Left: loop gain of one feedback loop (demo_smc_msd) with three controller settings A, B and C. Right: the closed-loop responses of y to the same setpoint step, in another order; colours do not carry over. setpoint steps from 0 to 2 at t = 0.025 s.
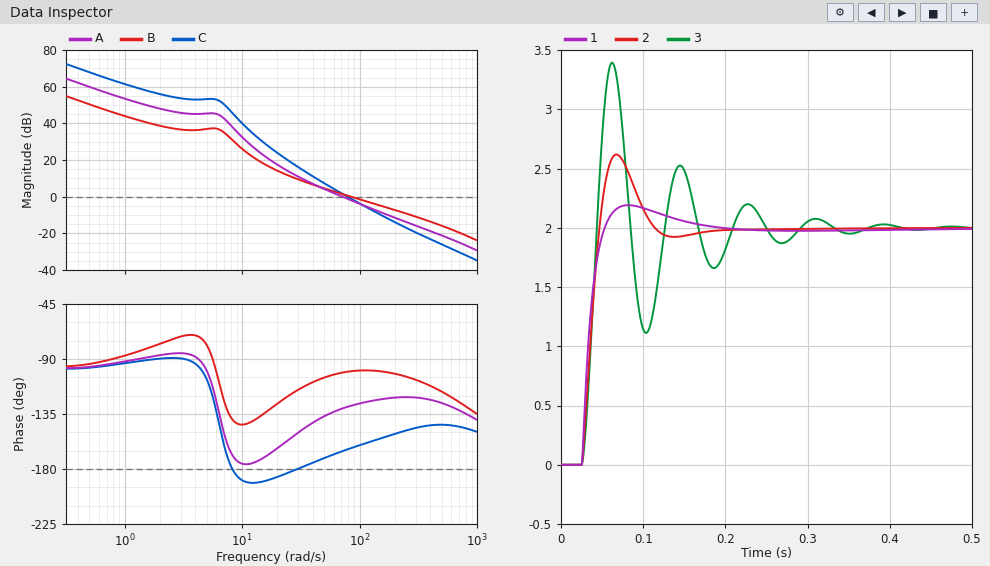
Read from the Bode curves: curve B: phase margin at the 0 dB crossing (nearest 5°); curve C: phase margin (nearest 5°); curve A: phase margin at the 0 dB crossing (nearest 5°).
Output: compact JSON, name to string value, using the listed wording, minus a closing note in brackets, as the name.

{"curve B: phase margin at the 0 dB crossing": "80°", "curve C: phase margin": "15°", "curve A: phase margin at the 0 dB crossing": "50°"}
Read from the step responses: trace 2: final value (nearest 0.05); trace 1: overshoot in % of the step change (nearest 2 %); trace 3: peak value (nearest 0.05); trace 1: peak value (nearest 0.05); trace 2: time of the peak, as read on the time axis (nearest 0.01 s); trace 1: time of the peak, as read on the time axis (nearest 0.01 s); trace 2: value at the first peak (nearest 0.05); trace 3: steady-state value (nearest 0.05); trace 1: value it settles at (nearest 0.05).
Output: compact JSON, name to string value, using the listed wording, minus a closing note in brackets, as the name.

{"trace 2: final value": "2.00", "trace 1: overshoot in % of the step change": "10 %", "trace 3: peak value": "3.40", "trace 1: peak value": "2.20", "trace 2: time of the peak, as read on the time axis": "0.07 s", "trace 1: time of the peak, as read on the time axis": "0.08 s", "trace 2: value at the first peak": "2.60", "trace 3: steady-state value": "2.00", "trace 1: value it settles at": "2.00"}
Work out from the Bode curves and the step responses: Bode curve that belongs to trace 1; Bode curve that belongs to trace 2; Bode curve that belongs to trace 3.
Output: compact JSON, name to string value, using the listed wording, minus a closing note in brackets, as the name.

{"Bode curve that belongs to trace 1": "B", "Bode curve that belongs to trace 2": "A", "Bode curve that belongs to trace 3": "C"}
